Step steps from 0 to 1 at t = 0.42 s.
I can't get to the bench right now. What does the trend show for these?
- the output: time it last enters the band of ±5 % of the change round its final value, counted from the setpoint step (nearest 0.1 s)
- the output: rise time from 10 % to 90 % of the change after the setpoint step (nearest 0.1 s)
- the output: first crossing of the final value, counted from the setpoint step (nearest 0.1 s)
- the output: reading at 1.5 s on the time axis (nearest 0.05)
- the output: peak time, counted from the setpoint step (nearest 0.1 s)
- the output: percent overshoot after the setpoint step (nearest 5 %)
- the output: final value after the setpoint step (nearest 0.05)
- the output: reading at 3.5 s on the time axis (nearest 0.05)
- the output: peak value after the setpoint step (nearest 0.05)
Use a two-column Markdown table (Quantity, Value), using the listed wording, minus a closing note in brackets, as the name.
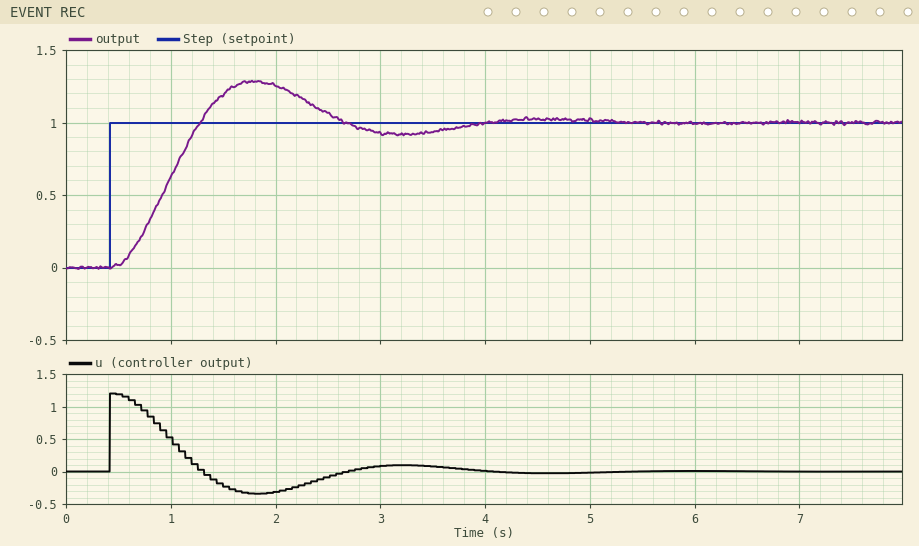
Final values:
| Quantity | Value |
|---|---|
| the output: time it last enters the band of ±5 % of the change round its final value, counted from the setpoint step | 3.2 s |
| the output: rise time from 10 % to 90 % of the change after the setpoint step | 0.6 s |
| the output: first crossing of the final value, counted from the setpoint step | 0.9 s |
| the output: reading at 1.5 s on the time axis | 1.20 |
| the output: peak time, counted from the setpoint step | 1.4 s |
| the output: percent overshoot after the setpoint step | 30 % |
| the output: final value after the setpoint step | 1.00 |
| the output: reading at 3.5 s on the time axis | 0.95 |
| the output: peak value after the setpoint step | 1.30 |
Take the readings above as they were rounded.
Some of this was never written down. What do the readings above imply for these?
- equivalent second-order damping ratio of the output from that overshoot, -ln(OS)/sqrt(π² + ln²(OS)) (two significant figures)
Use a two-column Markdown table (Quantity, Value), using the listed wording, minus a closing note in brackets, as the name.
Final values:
| Quantity | Value |
|---|---|
| equivalent second-order damping ratio of the output from that overshoot, -ln(OS)/sqrt(π² + ln²(OS)) | 0.36 |
